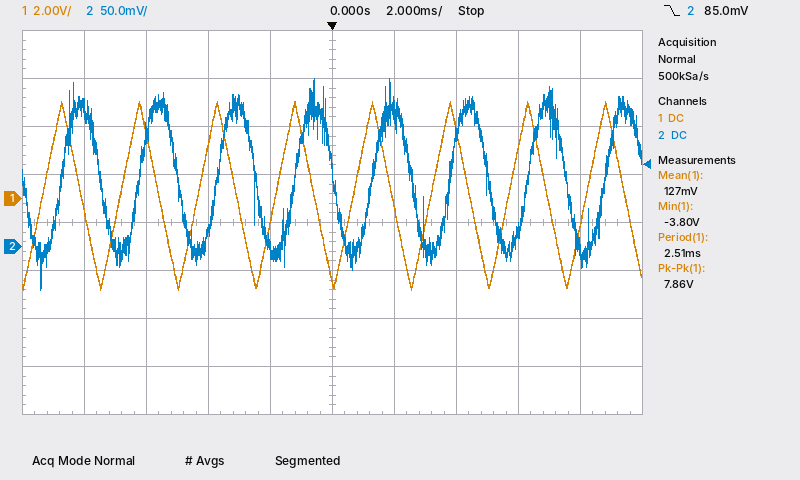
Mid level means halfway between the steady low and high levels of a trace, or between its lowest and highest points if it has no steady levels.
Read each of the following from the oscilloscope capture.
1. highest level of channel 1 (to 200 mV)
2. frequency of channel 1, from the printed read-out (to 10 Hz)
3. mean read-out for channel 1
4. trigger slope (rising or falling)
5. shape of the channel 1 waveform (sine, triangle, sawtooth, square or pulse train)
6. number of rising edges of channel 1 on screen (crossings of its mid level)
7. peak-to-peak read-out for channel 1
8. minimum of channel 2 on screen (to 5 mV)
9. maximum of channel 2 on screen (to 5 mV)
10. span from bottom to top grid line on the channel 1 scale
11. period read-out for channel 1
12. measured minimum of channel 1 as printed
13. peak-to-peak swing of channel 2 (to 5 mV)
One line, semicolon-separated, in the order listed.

4.0 V; 400 Hz; 127 mV; falling; triangle; 8; 7.86 V; -45 mV; 175 mV; 16 V; 2.51 ms; -3.80 V; 220 mV
